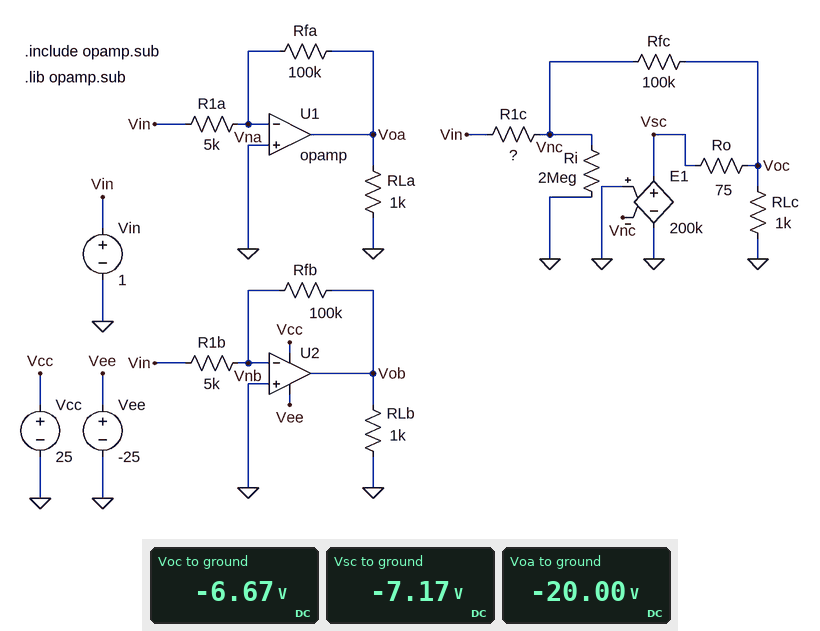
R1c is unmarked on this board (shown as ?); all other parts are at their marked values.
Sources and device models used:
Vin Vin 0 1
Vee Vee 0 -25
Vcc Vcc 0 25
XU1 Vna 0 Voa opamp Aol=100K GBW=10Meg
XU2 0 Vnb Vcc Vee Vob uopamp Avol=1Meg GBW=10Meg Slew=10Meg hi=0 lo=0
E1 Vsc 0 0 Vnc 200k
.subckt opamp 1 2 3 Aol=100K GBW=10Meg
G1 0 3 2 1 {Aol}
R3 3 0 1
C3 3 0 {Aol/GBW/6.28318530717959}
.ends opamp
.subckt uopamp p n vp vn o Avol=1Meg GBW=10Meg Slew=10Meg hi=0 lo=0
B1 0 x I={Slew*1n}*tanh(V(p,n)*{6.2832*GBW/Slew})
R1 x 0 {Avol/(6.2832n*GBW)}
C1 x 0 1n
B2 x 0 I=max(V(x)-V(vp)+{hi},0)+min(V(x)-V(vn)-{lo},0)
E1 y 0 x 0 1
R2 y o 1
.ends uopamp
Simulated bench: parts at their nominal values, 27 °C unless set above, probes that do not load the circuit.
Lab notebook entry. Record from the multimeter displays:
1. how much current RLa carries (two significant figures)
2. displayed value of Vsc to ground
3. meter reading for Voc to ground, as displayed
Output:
20 mA
-7.17 V
-6.67 V
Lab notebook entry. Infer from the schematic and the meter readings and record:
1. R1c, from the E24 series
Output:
15 kΩ
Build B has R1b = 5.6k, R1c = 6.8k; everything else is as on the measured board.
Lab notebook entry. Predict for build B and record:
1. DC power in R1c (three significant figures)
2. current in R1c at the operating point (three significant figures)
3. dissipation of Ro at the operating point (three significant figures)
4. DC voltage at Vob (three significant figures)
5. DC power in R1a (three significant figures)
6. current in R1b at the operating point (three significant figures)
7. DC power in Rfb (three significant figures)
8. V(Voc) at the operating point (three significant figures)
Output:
147 µW
147 µA
16.5 mW
-17.9 V
200 µW
179 µA
3.19 mW
-14.7 V
